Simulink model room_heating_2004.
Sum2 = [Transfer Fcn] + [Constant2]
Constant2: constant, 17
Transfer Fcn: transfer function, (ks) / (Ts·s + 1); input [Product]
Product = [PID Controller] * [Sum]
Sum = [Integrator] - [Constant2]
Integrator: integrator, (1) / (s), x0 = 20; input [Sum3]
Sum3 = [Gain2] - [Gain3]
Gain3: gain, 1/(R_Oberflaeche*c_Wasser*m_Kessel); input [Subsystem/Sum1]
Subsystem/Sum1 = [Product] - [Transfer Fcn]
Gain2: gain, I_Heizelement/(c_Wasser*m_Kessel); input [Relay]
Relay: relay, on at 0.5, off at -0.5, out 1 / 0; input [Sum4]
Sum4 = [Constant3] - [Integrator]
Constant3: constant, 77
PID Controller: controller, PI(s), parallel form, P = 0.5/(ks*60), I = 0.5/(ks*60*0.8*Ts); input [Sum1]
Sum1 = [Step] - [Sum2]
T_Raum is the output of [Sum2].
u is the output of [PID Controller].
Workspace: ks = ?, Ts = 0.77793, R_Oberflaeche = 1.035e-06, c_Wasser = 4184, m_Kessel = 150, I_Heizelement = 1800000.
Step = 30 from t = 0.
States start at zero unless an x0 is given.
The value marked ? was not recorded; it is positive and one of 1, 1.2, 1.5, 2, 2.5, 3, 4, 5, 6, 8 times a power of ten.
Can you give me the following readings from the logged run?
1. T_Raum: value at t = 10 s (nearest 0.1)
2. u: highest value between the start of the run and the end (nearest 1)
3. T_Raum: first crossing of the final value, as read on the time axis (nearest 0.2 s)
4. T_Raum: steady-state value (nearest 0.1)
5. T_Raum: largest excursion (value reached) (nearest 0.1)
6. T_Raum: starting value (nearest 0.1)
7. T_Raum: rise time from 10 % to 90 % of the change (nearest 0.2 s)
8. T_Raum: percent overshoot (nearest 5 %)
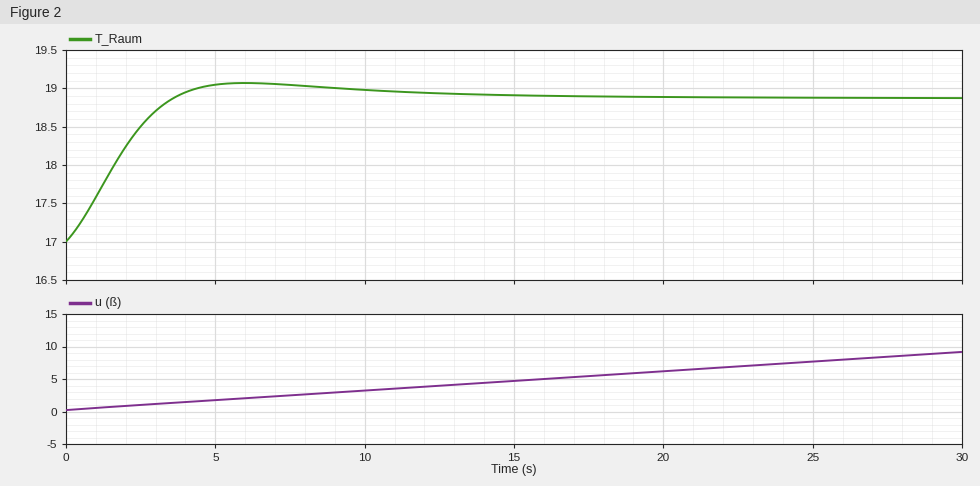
19.0
9
3.6 s
18.9
19.1
17.0
2.6 s
10 %
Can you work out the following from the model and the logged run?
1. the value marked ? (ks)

0.5
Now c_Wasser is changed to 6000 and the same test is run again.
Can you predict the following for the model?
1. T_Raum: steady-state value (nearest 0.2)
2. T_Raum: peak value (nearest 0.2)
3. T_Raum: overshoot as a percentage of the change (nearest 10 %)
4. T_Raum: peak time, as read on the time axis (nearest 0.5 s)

18.8
19.2
20 %
6.0 s
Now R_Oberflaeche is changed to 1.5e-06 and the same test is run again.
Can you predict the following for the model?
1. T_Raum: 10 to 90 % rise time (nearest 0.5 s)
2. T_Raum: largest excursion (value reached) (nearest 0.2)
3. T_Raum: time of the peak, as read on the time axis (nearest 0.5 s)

3.0 s
20.0
7.0 s
